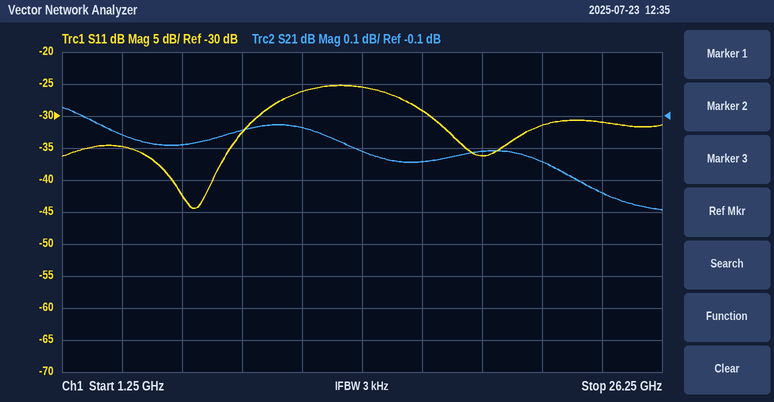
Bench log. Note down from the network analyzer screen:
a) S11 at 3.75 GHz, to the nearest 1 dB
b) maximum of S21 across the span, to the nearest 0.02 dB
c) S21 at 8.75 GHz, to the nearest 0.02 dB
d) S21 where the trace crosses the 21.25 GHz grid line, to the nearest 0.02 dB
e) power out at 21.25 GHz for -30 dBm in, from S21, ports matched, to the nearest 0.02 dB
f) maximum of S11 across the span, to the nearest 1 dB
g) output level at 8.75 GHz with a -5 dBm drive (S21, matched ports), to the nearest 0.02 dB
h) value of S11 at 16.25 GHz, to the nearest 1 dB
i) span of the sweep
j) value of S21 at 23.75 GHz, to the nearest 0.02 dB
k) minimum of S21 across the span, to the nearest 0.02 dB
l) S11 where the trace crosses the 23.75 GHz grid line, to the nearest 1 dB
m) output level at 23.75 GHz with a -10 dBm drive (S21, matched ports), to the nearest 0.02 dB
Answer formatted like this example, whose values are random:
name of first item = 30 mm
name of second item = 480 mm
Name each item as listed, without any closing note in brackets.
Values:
S11 at 3.75 GHz, to the nearest 1 dB = -35 dB
maximum of S21 across the span, to the nearest 0.02 dB = -0.08 dB
S21 at 8.75 GHz, to the nearest 0.02 dB = -0.14 dB
S21 where the trace crosses the 21.25 GHz grid line, to the nearest 0.02 dB = -0.24 dB
power out at 21.25 GHz for -30 dBm in, from S21, ports matched, to the nearest 0.02 dB = -30.24 dBm
maximum of S11 across the span, to the nearest 1 dB = -25 dB
output level at 8.75 GHz with a -5 dBm drive (S21, matched ports), to the nearest 0.02 dB = -5.14 dBm
value of S11 at 16.25 GHz, to the nearest 1 dB = -29 dB
span of the sweep = 25 GHz
value of S21 at 23.75 GHz, to the nearest 0.02 dB = -0.34 dB
minimum of S21 across the span, to the nearest 0.02 dB = -0.40 dB
S11 where the trace crosses the 23.75 GHz grid line, to the nearest 1 dB = -31 dB
output level at 23.75 GHz with a -10 dBm drive (S21, matched ports), to the nearest 0.02 dB = -10.34 dBm
